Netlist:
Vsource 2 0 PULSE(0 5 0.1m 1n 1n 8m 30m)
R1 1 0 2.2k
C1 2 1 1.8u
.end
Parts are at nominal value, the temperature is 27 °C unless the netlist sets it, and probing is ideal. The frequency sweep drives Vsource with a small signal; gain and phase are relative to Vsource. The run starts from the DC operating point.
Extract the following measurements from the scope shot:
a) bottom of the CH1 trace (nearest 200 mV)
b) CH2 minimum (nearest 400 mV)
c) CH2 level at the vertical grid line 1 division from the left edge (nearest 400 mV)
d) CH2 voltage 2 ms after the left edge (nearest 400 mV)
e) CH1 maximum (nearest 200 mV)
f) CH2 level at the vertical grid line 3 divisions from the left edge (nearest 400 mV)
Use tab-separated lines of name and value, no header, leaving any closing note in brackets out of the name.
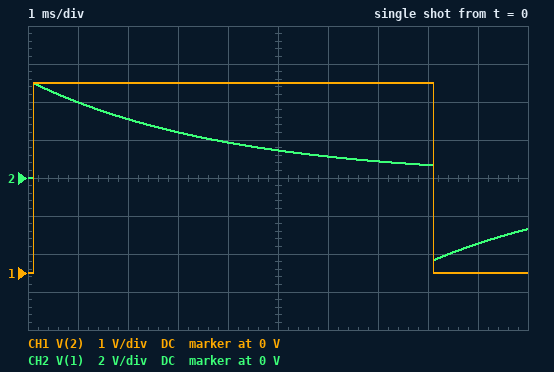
bottom of the CH1 trace	0 V
CH2 minimum	-4.4 V
CH2 level at the vertical grid line 1 division from the left edge	4.0 V
CH2 voltage 2 ms after the left edge	3.2 V
CH1 maximum	5.0 V
CH2 level at the vertical grid line 3 divisions from the left edge	2.4 V
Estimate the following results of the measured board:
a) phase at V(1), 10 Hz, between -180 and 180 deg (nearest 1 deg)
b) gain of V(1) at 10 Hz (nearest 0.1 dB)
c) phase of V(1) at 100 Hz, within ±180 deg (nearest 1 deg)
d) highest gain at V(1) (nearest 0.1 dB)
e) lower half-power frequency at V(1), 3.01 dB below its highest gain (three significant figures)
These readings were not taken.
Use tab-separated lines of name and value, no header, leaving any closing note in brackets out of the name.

phase at V(1), 10 Hz, between -180 and 180 deg	76 deg
gain of V(1) at 10 Hz	-12.3 dB
phase of V(1) at 100 Hz, within ±180 deg	22 deg
highest gain at V(1)	0 dB
lower half-power frequency at V(1), 3.01 dB below its highest gain	40.2 Hz
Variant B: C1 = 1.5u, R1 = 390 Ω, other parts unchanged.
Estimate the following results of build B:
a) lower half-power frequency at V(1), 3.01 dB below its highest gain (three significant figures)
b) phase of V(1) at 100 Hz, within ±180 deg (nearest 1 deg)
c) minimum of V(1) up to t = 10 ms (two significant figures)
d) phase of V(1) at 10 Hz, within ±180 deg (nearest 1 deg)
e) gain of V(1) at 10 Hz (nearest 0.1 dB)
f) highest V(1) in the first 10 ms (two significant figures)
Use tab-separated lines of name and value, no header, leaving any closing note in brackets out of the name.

lower half-power frequency at V(1), 3.01 dB below its highest gain	272 Hz
phase of V(1) at 100 Hz, within ±180 deg	70 deg
minimum of V(1) up to t = 10 ms	-5.0 V
phase of V(1) at 10 Hz, within ±180 deg	88 deg
gain of V(1) at 10 Hz	-28.7 dB
highest V(1) in the first 10 ms	5.0 V
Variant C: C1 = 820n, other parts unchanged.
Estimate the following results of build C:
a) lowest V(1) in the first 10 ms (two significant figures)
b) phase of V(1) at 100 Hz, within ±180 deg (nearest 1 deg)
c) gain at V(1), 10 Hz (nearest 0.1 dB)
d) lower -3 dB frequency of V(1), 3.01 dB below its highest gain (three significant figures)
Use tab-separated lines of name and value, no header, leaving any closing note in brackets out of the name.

lowest V(1) in the first 10 ms	-4.9 V
phase of V(1) at 100 Hz, within ±180 deg	41 deg
gain at V(1), 10 Hz	-19.0 dB
lower -3 dB frequency of V(1), 3.01 dB below its highest gain	88.2 Hz
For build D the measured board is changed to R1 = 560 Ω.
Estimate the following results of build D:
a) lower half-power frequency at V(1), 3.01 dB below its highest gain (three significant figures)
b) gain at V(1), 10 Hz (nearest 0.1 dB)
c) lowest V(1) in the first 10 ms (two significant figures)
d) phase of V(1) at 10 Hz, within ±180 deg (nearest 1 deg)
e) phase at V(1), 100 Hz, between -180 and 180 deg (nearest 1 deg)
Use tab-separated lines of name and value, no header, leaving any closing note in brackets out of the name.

lower half-power frequency at V(1), 3.01 dB below its highest gain	158 Hz
gain at V(1), 10 Hz	-24.0 dB
lowest V(1) in the first 10 ms	-5.0 V
phase of V(1) at 10 Hz, within ±180 deg	86 deg
phase at V(1), 100 Hz, between -180 and 180 deg	58 deg
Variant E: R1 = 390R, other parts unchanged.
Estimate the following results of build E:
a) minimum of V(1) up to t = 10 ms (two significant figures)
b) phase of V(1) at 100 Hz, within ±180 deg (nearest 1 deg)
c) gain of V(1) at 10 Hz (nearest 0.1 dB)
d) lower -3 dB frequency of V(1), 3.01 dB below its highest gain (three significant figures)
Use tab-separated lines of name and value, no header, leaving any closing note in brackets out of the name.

minimum of V(1) up to t = 10 ms	-5.0 V
phase of V(1) at 100 Hz, within ±180 deg	66 deg
gain of V(1) at 10 Hz	-27.1 dB
lower -3 dB frequency of V(1), 3.01 dB below its highest gain	227 Hz
